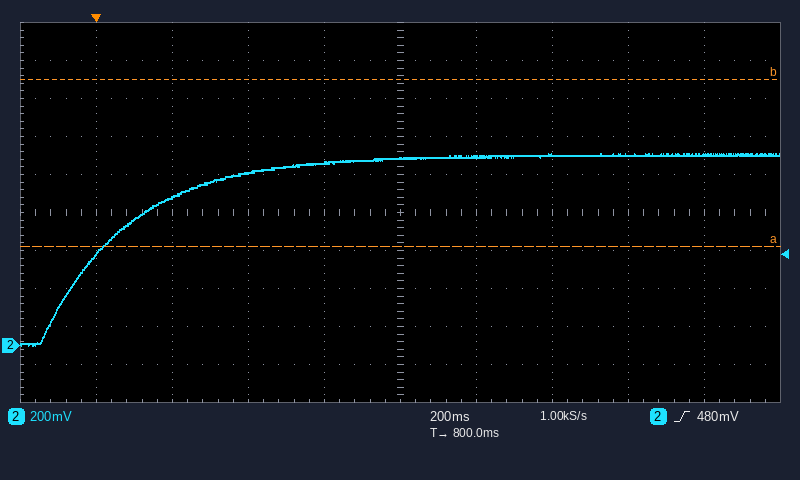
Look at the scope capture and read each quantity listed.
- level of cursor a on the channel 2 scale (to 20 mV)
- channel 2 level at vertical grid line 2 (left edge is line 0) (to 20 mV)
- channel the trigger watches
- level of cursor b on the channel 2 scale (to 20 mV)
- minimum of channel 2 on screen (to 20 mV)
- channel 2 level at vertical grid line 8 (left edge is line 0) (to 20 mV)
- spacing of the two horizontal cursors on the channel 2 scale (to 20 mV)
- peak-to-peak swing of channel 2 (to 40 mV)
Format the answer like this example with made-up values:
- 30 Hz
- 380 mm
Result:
- 520 mV
- 780 mV
- channel 2
- 1.40 V
- 0 mV
- 1.00 V
- 880 mV
- 1.00 V
